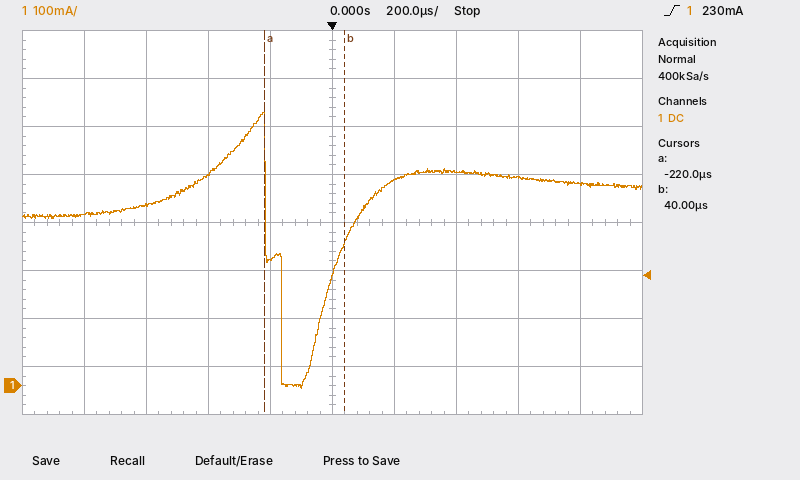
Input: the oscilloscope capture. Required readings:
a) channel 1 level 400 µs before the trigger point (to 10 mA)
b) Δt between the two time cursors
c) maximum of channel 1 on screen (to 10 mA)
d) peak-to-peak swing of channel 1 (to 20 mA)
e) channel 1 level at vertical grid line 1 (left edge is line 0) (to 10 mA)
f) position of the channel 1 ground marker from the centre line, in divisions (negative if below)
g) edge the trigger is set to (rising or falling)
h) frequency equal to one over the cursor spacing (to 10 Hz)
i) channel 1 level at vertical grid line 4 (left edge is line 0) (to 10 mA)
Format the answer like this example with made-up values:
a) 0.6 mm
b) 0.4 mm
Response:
a) 440 mA
b) 260 µs
c) 570 mA
d) 580 mA
e) 360 mA
f) -3.4 div
g) rising
h) 3.85 kHz
i) 260 mA
